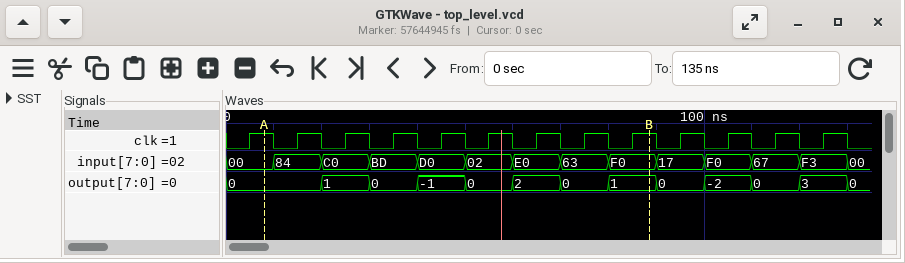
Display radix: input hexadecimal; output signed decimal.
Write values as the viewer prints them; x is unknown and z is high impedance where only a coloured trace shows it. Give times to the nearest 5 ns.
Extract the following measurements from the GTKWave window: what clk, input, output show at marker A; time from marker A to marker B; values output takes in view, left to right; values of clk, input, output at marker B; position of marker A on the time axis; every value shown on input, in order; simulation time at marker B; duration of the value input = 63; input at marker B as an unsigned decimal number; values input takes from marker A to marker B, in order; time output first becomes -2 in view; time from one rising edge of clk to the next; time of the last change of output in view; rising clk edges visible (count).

clk=1, input=00, output=0
80 ns
0, 1, 0, -1, 0, 2, 0, 1, 0, -2, 0, 3, 0
clk=1, input=F0, output=1
10 ns
00, 84, C0, BD, D0, 02, E0, 63, F0, 17, F0, 67, F3, 00
90 ns
10 ns
240
00, 84, C0, BD, D0, 02, E0, 63, F0
100 ns
10 ns
130 ns
13
